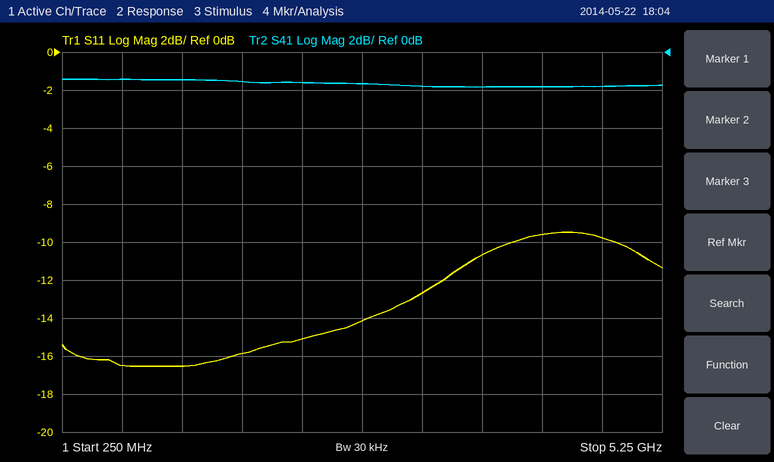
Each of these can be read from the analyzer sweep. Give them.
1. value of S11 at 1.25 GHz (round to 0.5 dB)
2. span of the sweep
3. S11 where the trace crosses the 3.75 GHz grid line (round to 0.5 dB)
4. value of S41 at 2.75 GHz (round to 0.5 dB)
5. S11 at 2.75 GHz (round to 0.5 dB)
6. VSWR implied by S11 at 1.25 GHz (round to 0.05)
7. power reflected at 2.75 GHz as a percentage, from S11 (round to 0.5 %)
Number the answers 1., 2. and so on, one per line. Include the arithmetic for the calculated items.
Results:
1. -16.5 dB
2. 5 GHz
3. -10.5 dB
4. -1.5 dB
5. -14.0 dB
6. |Γ| = 10^(-16.5/20) = 0.1496; VSWR = (1 + 0.1496)/(1 − 0.1496) ≈ 1.35
7. 10^(-14/10) ≈ 4.0 %
